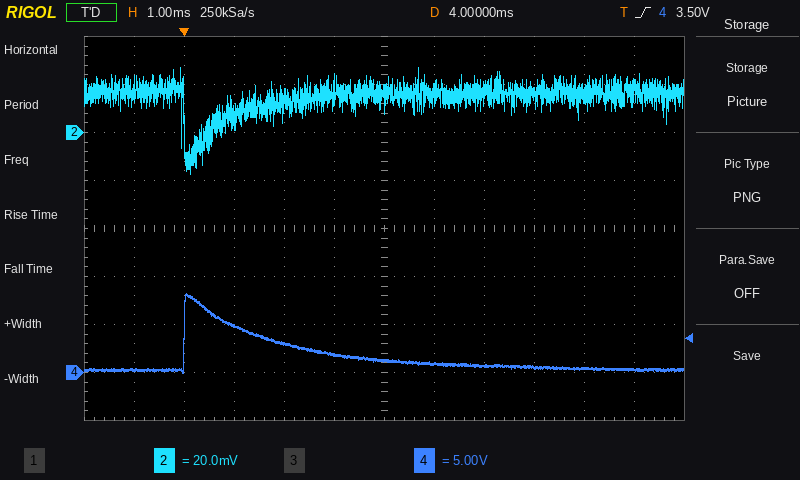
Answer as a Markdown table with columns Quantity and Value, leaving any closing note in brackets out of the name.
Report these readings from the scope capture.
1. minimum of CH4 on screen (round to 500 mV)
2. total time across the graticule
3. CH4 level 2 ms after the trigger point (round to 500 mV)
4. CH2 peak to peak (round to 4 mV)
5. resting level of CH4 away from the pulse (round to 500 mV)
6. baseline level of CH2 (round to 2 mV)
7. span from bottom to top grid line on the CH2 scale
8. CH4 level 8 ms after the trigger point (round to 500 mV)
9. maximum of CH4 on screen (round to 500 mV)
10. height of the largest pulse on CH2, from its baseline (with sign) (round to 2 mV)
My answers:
| Quantity | Value |
|---|---|
| minimum of CH4 on screen | 0.0 V |
| total time across the graticule | 12 ms |
| CH4 level 2 ms after the trigger point | 3.0 V |
| CH2 peak to peak | 44 mV |
| resting level of CH4 away from the pulse | 500 mV |
| baseline level of CH2 | 16 mV |
| span from bottom to top grid line on the CH2 scale | 160 mV |
| CH4 level 8 ms after the trigger point | 500 mV |
| maximum of CH4 on screen | 8.0 V |
| height of the largest pulse on CH2, from its baseline (with sign) | -34 mV |
